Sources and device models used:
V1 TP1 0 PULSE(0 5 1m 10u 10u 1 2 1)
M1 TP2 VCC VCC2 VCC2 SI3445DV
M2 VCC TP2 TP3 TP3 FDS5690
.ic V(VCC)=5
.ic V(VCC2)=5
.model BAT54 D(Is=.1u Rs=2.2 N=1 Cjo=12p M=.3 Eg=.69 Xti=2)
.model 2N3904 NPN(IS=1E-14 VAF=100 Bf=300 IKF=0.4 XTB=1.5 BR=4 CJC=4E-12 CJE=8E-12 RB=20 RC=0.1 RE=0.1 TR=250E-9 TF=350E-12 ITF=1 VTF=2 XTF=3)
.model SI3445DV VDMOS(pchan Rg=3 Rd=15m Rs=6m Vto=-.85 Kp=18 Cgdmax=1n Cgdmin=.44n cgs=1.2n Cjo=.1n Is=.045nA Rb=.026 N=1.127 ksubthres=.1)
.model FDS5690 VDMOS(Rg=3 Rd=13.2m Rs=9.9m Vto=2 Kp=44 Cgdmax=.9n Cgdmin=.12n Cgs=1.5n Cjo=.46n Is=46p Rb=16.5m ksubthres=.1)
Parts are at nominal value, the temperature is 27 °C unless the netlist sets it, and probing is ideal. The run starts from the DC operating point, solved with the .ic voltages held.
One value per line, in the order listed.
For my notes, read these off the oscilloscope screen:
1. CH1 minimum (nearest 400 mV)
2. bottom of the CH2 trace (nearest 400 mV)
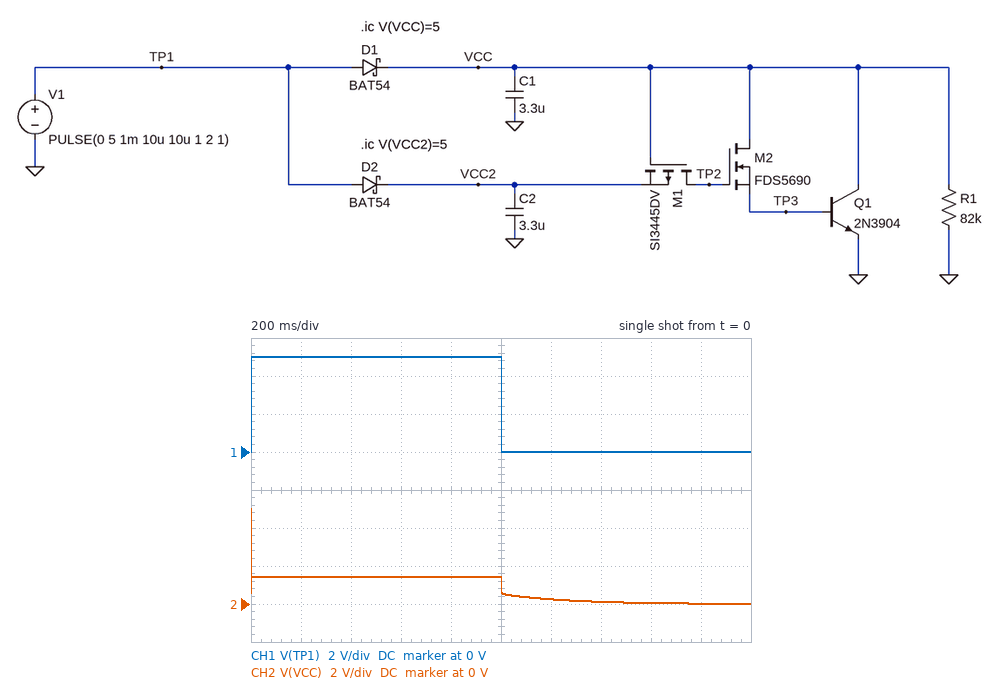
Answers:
0 V
0 V
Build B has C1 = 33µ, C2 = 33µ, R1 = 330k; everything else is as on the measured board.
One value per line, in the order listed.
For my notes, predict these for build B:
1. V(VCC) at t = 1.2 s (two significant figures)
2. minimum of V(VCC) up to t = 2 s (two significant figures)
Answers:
510 mV
450 mV
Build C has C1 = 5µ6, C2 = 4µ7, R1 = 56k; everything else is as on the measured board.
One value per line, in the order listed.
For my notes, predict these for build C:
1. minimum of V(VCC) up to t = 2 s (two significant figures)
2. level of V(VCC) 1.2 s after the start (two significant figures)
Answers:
18 mV
280 mV
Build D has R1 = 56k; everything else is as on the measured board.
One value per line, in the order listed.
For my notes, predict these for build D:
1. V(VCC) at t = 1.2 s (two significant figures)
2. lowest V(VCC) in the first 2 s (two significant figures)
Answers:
180 mV
1.3 mV
